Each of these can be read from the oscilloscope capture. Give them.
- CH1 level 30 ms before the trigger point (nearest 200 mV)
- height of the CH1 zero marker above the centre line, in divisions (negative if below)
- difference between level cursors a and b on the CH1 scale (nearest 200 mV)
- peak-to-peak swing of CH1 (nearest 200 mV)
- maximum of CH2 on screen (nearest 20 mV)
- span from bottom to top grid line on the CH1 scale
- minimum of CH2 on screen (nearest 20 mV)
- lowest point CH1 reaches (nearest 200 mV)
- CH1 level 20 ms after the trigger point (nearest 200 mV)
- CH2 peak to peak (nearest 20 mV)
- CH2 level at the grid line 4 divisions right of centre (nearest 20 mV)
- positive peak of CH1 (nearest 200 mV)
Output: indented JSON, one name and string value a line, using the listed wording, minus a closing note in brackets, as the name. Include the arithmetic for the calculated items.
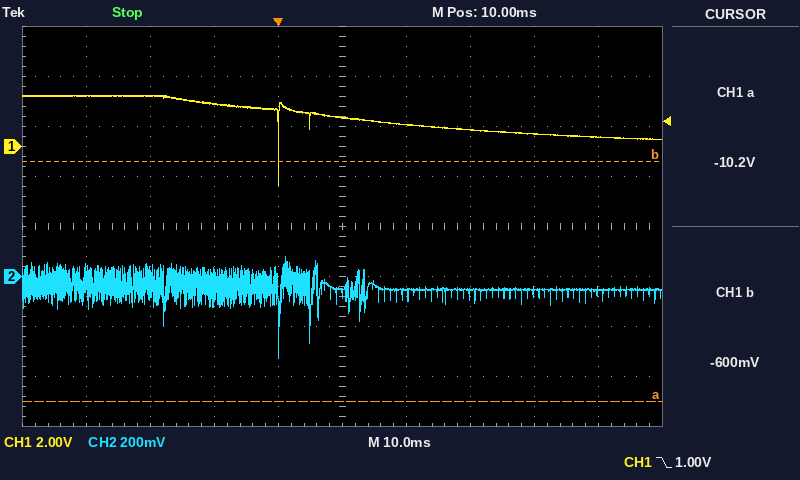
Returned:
{
  "CH1 level 30 ms before the trigger point": "2.0 V",
  "height of the CH1 zero marker above the centre line, in divisions": "+1.6 div",
  "difference between level cursors a and b on the CH1 scale": "9.6 V",
  "peak-to-peak swing of CH1": "2.0 V − (-1.6 V) = 3.6 V",
  "maximum of CH2 on screen": "80 mV",
  "span from bottom to top grid line on the CH1 scale": "16 V",
  "minimum of CH2 on screen": "-320 mV",
  "lowest point CH1 reaches": "-1.6 V",
  "CH1 level 20 ms after the trigger point": "800 mV",
  "CH2 peak to peak": "80 mV − (-320 mV) = 400 mV",
  "CH2 level at the grid line 4 divisions right of centre": "-60 mV",
  "positive peak of CH1": "2.0 V"
}
